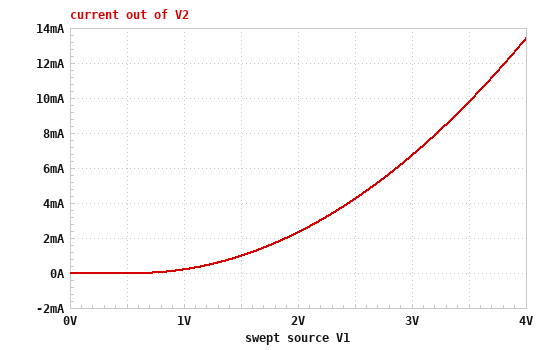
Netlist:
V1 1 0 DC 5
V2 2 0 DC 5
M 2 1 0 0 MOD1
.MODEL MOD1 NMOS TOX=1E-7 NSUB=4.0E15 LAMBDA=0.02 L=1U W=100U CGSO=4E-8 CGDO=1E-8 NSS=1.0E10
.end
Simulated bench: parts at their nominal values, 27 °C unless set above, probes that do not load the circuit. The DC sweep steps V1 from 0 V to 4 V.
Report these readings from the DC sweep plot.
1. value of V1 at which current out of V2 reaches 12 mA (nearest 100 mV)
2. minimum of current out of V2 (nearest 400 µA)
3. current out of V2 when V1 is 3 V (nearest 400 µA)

3.8 V
0 A
6.8 mA
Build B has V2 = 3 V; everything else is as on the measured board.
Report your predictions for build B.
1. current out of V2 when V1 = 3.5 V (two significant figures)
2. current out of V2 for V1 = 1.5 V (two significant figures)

9.4 mA
950 µA
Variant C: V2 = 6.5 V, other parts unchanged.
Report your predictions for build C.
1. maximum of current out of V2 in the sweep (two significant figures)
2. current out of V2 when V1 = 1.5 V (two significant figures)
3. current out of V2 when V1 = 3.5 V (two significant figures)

14 mA
1.0 mA
10 mA
